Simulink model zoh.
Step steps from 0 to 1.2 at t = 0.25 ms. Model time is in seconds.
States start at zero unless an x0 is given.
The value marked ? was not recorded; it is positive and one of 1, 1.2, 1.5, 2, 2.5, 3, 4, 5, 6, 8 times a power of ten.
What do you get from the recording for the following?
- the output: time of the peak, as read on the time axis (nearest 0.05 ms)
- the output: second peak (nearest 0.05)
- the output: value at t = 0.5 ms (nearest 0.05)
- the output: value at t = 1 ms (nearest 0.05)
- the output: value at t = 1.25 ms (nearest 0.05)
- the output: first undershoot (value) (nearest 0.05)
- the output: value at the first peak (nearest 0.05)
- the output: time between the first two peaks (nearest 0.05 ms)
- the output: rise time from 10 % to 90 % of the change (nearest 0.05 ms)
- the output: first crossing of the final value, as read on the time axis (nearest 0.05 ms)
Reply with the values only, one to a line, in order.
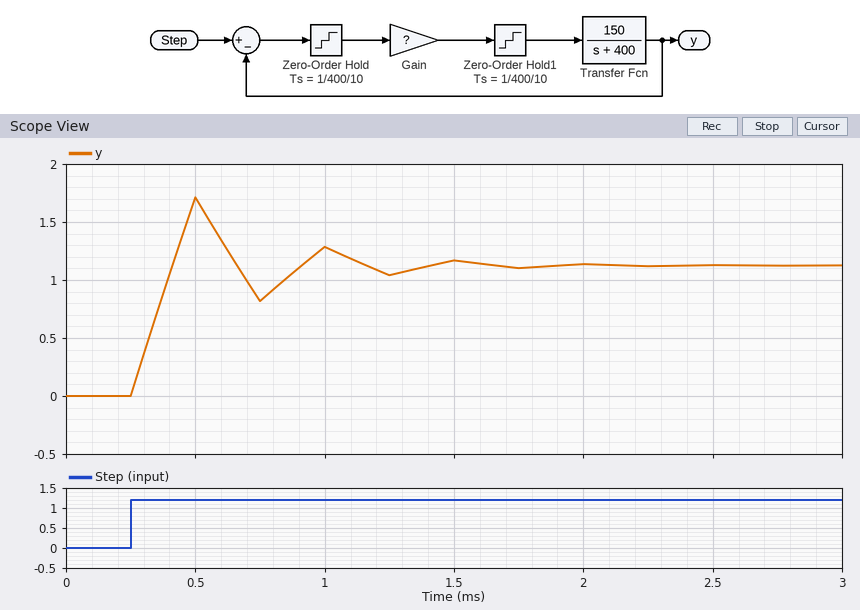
0.50 ms
1.30
1.70
1.30
1.05
0.80
1.70
0.50 ms
0.15 ms
0.40 ms
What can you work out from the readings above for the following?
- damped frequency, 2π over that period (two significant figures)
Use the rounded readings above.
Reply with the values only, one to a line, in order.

13 rad/ms
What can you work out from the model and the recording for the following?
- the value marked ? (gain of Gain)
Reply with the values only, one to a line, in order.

40
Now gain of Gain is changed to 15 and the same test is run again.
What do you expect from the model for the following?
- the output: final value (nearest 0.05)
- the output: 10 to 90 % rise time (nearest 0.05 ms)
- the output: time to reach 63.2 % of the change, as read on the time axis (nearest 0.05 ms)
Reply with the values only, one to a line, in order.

1.00
0.55 ms
0.50 ms
